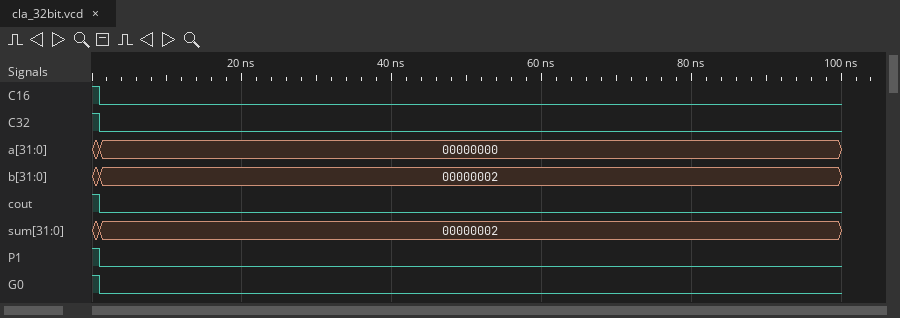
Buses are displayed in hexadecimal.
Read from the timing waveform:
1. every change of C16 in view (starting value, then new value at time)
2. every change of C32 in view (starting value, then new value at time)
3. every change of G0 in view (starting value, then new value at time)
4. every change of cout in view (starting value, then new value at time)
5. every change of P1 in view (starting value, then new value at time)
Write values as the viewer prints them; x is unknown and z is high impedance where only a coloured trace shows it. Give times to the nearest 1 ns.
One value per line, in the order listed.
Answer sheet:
1, 0 at 1 ns
1, 0 at 1 ns
1, 0 at 1 ns
1, 0 at 1 ns
1, 0 at 1 ns
